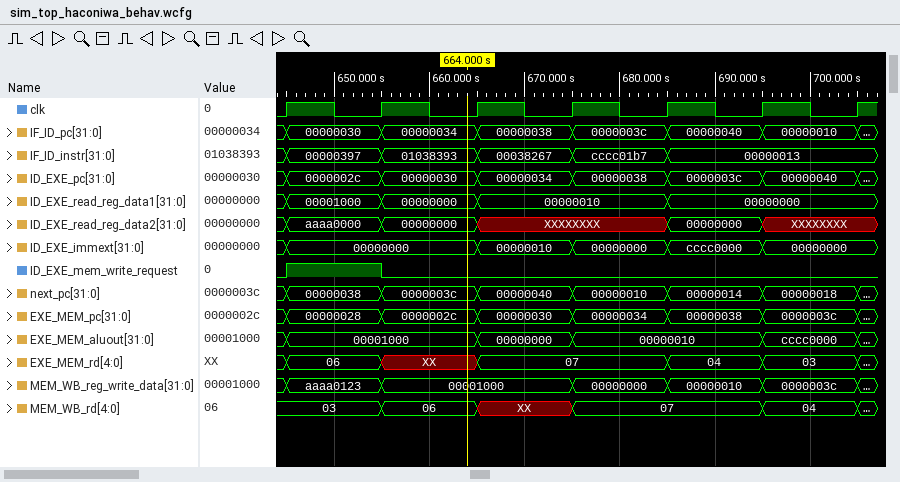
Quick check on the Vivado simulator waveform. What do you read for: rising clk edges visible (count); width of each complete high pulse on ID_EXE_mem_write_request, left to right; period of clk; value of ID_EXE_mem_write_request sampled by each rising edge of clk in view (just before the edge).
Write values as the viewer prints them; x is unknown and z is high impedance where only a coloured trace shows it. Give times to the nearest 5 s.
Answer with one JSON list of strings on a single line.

["7", "10 s", "10 s", "0 1 0 0 0 0 0"]
